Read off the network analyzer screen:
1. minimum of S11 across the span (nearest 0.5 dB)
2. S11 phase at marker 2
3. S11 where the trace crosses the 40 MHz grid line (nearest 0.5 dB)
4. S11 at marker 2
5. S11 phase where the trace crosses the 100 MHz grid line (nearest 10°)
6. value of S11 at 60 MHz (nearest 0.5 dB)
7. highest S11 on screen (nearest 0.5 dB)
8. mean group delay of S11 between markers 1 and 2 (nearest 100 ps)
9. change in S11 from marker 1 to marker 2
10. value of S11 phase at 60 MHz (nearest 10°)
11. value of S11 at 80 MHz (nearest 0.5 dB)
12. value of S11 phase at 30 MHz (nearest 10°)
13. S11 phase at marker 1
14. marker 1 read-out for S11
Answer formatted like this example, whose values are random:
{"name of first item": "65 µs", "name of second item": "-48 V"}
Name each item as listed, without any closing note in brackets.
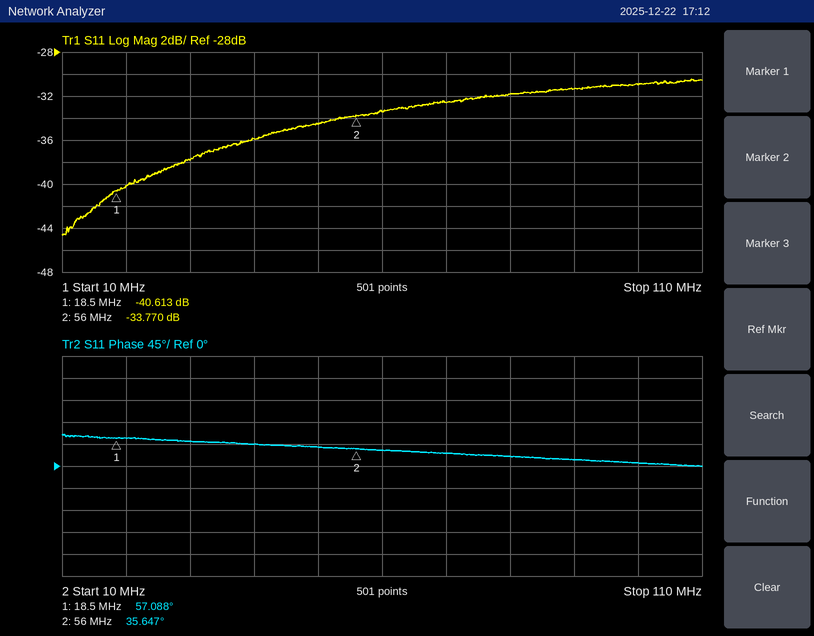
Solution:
{"minimum of S11 across the span": "-44.5 dB", "S11 phase at marker 2": "35.647°", "S11 where the trace crosses the 40 MHz grid line": "-36.0 dB", "S11 at marker 2": "-33.770 dB", "S11 phase where the trace crosses the 100 MHz grid line": "10°", "value of S11 at 60 MHz": "-33.5 dB", "highest S11 on screen": "-30.5 dB", "mean group delay of S11 between markers 1 and 2": "1.6 ns", "change in S11 from marker 1 to marker 2": "6.843 dB", "value of S11 phase at 60 MHz": "30°", "value of S11 at 80 MHz": "-32.0 dB", "value of S11 phase at 30 MHz": "50°", "S11 phase at marker 1": "57.088°", "marker 1 read-out for S11": "-40.613 dB"}
